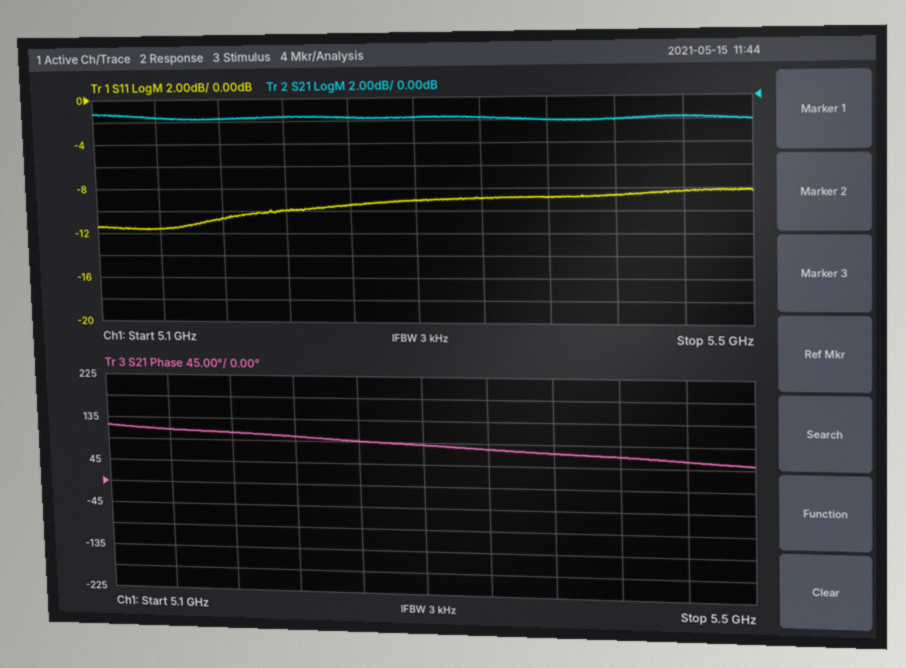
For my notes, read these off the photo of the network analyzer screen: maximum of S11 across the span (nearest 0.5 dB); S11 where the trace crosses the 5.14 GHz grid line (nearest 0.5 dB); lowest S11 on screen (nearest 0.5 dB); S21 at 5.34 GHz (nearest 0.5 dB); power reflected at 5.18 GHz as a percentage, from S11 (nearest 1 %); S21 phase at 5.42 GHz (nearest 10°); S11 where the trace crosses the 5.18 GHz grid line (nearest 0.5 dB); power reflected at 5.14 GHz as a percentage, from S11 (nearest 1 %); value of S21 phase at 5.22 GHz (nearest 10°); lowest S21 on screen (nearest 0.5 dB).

-8.0 dB
-11.5 dB
-11.5 dB
-2.0 dB
9 %
70°
-10.5 dB
7 %
100°
-2.0 dB
